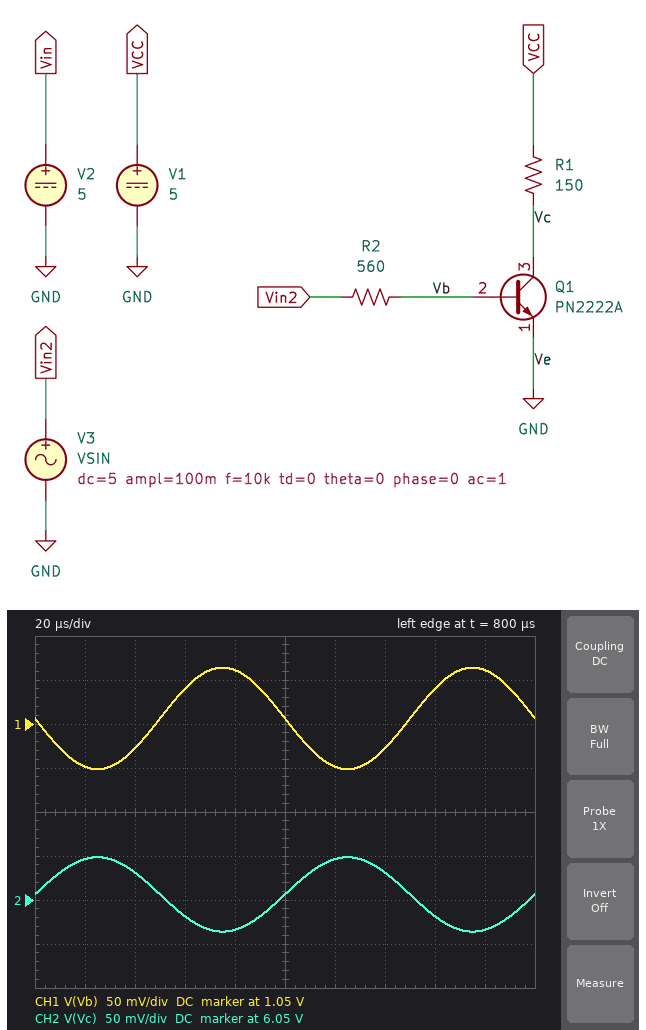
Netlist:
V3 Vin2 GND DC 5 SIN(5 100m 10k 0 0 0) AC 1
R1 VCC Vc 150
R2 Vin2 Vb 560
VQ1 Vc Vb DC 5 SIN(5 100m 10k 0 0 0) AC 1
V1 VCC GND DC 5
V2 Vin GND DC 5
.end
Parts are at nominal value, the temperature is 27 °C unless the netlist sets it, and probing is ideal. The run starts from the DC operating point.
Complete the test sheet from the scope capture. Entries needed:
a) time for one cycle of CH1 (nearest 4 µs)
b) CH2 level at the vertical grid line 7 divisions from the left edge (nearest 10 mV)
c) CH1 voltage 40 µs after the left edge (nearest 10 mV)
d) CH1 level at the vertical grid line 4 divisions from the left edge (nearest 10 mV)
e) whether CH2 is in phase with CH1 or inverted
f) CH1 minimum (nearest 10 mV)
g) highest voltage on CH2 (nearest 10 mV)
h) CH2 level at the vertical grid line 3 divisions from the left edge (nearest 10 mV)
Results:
100 µs
6.08 V
1.02 V
1.11 V
inverted
1.00 V
6.10 V
6.03 V
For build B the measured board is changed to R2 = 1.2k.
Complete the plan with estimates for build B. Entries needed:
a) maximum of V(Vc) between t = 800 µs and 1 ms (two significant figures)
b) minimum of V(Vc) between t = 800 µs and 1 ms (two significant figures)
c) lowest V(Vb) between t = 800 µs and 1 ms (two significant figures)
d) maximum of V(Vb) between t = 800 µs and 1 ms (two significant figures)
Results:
5.6 V
5.5 V
480 mV
630 mV
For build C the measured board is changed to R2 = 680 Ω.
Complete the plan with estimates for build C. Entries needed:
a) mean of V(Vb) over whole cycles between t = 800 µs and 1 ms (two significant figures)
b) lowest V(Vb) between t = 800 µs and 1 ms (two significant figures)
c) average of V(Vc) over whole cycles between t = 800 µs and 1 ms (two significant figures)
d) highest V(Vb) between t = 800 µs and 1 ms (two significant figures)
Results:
900 mV
840 mV
5.9 V
970 mV
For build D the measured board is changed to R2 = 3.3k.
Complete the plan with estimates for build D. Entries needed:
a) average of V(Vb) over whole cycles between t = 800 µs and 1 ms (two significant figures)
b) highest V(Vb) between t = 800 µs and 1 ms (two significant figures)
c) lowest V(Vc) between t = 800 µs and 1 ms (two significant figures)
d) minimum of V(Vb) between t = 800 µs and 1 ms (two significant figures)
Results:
220 mV
310 mV
5.2 V
130 mV
